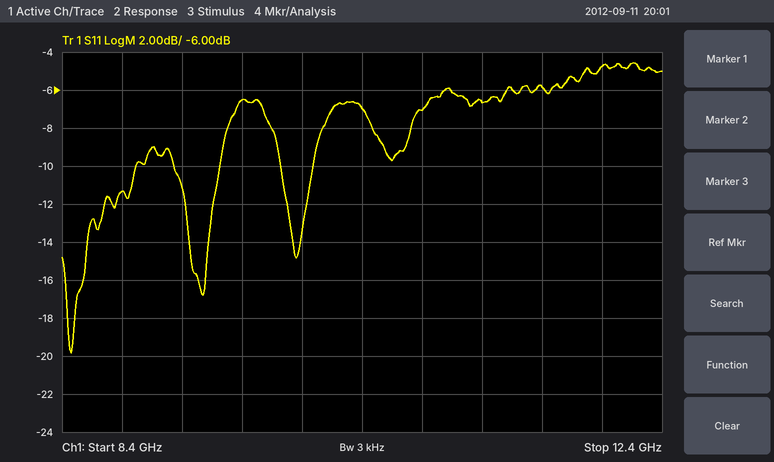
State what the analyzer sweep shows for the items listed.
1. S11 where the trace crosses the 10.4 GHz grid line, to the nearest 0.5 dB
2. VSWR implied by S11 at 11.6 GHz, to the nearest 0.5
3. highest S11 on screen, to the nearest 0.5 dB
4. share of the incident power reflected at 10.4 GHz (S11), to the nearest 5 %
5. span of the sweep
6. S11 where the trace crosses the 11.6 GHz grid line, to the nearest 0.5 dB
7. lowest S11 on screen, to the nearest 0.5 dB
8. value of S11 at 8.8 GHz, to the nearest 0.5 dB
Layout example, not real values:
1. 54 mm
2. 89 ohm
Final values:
1. -7.0 dB
2. 3.0
3. -4.5 dB
4. 20 %
5. 4 GHz
6. -6.0 dB
7. -20.0 dB
8. -11.5 dB
